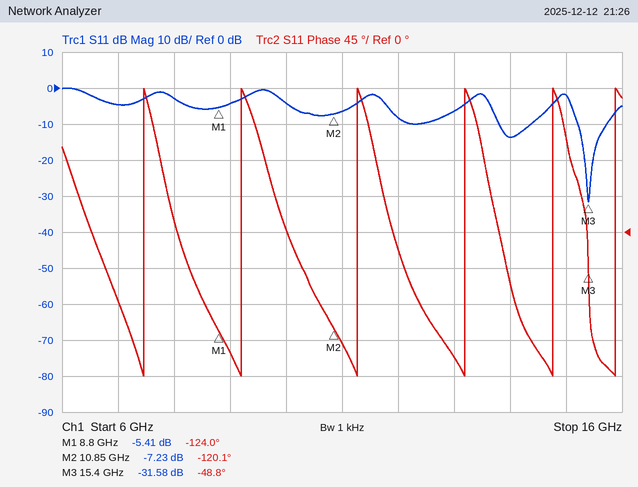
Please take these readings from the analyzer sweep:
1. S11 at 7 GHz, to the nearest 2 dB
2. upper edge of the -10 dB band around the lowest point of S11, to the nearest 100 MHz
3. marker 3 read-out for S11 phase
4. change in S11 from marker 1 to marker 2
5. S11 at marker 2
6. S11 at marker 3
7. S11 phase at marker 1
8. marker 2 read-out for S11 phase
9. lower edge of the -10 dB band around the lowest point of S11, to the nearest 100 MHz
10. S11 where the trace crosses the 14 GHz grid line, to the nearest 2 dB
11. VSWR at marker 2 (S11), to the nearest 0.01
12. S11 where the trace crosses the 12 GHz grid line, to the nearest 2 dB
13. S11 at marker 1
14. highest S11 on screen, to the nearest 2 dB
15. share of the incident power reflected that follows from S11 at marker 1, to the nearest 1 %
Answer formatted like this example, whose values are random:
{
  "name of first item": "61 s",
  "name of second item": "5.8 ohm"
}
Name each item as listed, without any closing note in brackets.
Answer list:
{
  "S11 at 7 GHz, to the nearest 2 dB": "-4 dB",
  "upper edge of the -10 dB band around the lowest point of S11, to the nearest 100 MHz": "15.7 GHz",
  "marker 3 read-out for S11 phase": "-48.8°",
  "change in S11 from marker 1 to marker 2": "-1.82 dB",
  "S11 at marker 2": "-7.23 dB",
  "S11 at marker 3": "-31.58 dB",
  "S11 phase at marker 1": "-124.0°",
  "marker 2 read-out for S11 phase": "-120.1°",
  "lower edge of the -10 dB band around the lowest point of S11, to the nearest 100 MHz": "15.2 GHz",
  "S11 where the trace crosses the 14 GHz grid line, to the nearest 2 dB": "-14 dB",
  "VSWR at marker 2 (S11), to the nearest 0.01": "2.54",
  "S11 where the trace crosses the 12 GHz grid line, to the nearest 2 dB": "-8 dB",
  "S11 at marker 1": "-5.41 dB",
  "highest S11 on screen, to the nearest 2 dB": "0 dB",
  "share of the incident power reflected that follows from S11 at marker 1, to the nearest 1 %": "29 %"
}
